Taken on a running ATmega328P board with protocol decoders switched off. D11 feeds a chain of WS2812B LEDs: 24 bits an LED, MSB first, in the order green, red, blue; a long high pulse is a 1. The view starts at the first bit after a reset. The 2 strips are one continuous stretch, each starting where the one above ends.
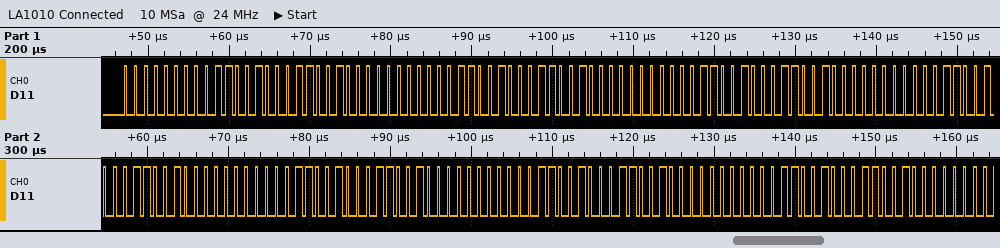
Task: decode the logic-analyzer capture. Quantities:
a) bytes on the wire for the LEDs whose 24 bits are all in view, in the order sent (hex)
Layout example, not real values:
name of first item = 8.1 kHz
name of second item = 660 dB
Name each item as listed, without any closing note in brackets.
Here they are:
bytes on the wire for the LEDs whose 24 bits are all in view, in the order sent = 00 64 64 00 64 64 00 64 64 00 64 64 00 64 64 00 64 64 00 64 64
